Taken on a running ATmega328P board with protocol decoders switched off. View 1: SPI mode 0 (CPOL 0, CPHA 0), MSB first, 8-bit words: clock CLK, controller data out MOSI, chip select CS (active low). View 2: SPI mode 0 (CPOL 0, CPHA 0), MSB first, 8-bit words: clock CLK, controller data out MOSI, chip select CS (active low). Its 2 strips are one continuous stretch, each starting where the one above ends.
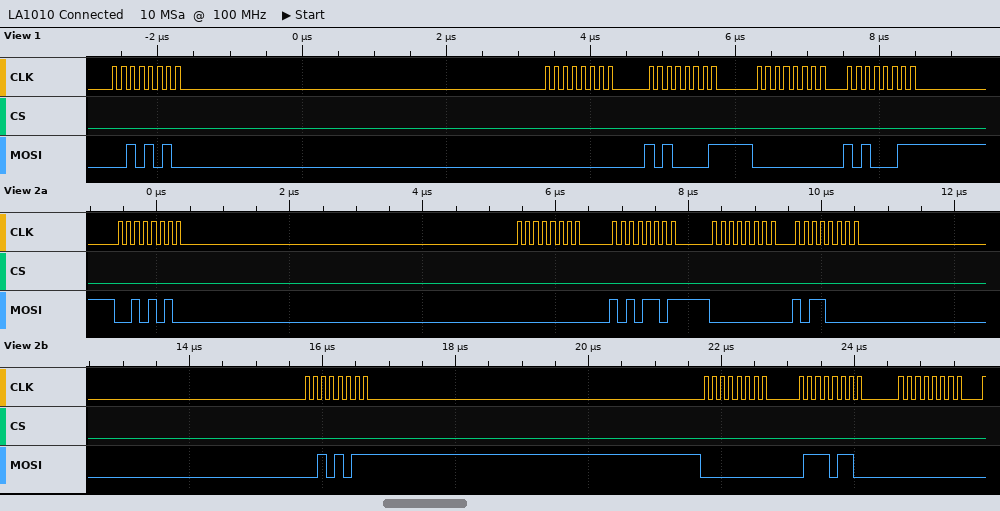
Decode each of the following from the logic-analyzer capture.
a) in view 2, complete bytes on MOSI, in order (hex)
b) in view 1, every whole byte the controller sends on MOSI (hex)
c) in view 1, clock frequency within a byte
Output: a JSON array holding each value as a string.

["0x2A 0x00 0xAD 0x00 0xB0 0x2B 0x00 0x76 0x00", "2A 00 A1 00 A3", "8 MHz"]
